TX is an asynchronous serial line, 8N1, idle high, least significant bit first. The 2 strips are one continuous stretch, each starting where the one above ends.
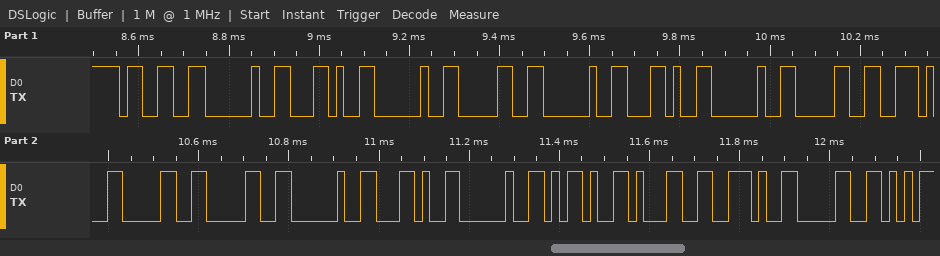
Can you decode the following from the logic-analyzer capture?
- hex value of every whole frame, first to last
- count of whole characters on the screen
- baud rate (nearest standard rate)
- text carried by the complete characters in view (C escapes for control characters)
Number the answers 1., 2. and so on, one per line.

1. 33 20 2C 20 30 20 2C 20 30 2E 30 30 20 2C 20 2D 31 2E 30
2. 19
3. 57600 baud
4. "3 , 0 , 0.00 , -1.0"
